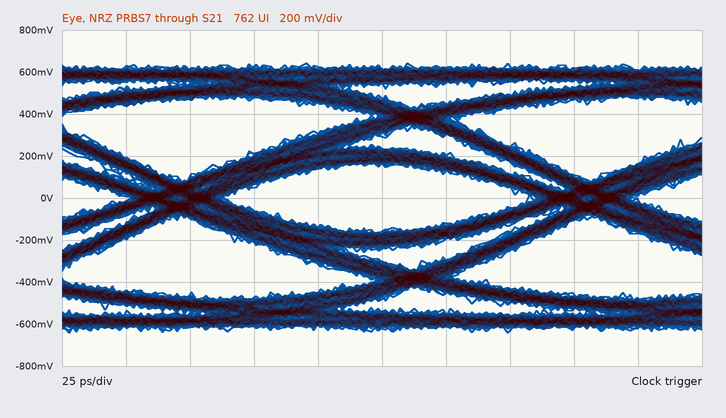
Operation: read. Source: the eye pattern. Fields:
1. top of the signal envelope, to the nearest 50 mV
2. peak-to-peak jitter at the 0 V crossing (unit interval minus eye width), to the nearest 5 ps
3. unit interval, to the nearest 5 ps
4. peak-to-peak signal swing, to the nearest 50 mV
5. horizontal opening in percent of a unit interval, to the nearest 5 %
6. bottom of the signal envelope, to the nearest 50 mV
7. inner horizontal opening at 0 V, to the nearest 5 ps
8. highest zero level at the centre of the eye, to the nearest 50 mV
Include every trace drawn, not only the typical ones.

650 mV
40 ps
160 ps
1.30 V
75 %
-650 mV
120 ps
-150 mV
